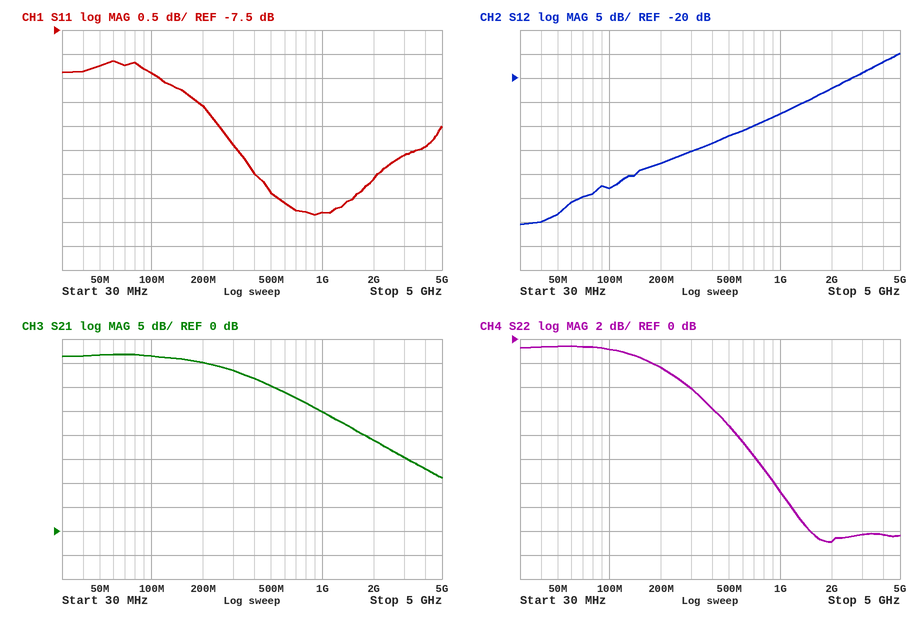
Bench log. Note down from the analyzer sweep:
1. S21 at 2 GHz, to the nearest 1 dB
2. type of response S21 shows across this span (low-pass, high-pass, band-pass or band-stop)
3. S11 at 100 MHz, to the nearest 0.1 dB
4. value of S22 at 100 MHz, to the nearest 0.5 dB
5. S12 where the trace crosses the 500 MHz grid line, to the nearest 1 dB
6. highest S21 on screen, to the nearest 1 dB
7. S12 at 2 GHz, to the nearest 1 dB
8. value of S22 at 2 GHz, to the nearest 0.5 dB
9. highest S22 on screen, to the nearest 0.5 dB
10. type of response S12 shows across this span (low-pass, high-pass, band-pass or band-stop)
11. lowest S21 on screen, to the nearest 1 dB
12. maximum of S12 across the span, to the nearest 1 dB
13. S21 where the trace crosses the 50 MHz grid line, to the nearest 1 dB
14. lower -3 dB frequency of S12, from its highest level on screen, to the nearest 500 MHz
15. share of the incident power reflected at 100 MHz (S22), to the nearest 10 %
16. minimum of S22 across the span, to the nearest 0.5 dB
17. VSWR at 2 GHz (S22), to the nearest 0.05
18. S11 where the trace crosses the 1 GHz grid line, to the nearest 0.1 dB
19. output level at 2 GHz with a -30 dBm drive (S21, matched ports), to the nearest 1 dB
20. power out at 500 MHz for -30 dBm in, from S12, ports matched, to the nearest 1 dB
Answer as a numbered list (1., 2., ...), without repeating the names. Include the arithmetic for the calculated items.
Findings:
1. 19 dB
2. low-pass
3. -8.4 dB
4. -1.0 dB
5. -32 dB
6. 37 dB
7. -22 dB
8. -17.0 dB
9. -0.5 dB
10. high-pass
11. 11 dB
12. -15 dB
13. 37 dB
14. 3.5 GHz
15. 10^(-1/10) ≈ 79.4 %, so 80 % to the nearest 10 %
16. -17.0 dB
17. |Γ| = 10^(-17/20) = 0.1413; VSWR = (1 + 0.1413)/(1 − 0.1413) ≈ 1.33, so 1.35 to the nearest 0.05
18. -11.3 dB
19. -30 dBm + (19 dB) = -11 dBm
20. -30 dBm + (-32 dB) = -62 dBm
